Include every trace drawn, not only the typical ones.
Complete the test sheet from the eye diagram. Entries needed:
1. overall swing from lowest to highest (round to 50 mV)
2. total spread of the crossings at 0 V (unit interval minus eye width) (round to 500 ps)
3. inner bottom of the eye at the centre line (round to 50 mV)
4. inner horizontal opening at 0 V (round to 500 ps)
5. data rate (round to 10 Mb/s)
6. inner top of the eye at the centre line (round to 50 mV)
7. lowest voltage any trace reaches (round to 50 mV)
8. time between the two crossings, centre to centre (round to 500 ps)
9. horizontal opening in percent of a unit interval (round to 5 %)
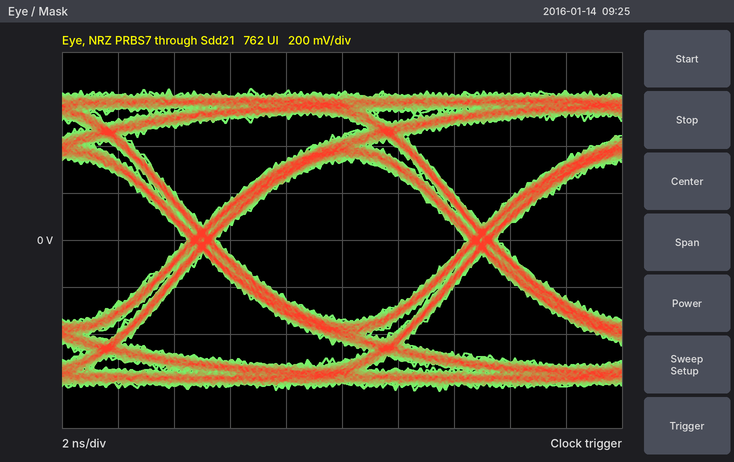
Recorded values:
1.30 V
1.0 ns
-350 mV
9.0 ns
100 Mb/s
350 mV
-650 mV
10.0 ns
90 %
